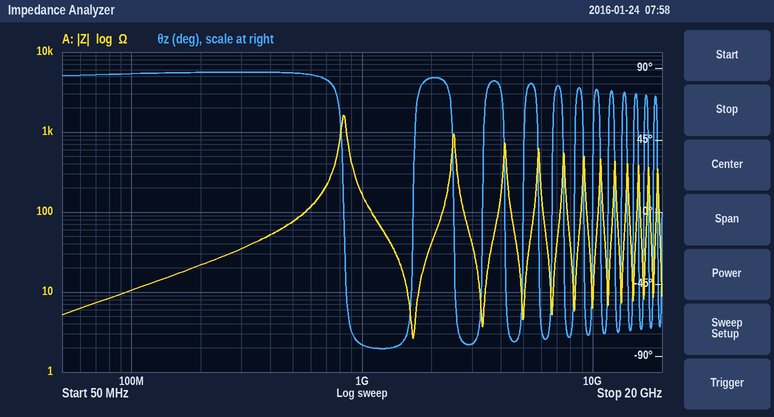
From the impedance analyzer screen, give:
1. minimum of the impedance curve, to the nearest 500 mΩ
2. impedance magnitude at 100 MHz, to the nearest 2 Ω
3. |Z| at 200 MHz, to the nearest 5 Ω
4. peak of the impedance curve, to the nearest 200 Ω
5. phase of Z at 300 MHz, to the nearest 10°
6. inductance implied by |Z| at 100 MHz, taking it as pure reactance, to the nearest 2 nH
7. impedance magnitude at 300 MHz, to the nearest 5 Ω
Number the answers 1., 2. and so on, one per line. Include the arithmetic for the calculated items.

1. 2.5 Ω
2. 10 Ω
3. 20 Ω
4. 1.6 kΩ
5. 90°
6. L = 10 Ω/(2π × 100 MHz) ≈ 16 nH
7. 35 Ω
